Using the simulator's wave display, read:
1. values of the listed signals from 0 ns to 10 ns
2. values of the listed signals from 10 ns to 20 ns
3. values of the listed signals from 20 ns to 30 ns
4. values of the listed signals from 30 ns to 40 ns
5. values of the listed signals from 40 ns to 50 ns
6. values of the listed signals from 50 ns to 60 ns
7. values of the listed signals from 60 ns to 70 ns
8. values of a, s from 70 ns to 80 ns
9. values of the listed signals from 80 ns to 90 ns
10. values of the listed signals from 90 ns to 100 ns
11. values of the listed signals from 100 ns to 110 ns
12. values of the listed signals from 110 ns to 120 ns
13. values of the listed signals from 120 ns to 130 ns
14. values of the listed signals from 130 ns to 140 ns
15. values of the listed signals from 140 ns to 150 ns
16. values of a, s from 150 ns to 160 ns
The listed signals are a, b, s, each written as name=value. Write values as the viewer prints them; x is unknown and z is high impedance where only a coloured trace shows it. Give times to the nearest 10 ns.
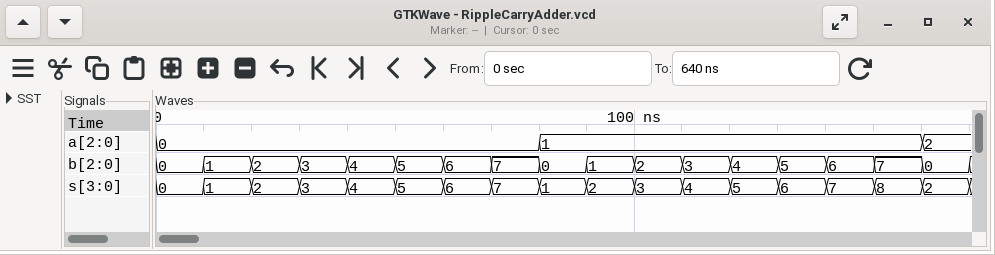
a=0, b=0, s=0
a=0, b=1, s=1
a=0, b=2, s=2
a=0, b=3, s=3
a=0, b=4, s=4
a=0, b=5, s=5
a=0, b=6, s=6
a=0, s=7
a=1, b=0, s=1
a=1, b=1, s=2
a=1, b=2, s=3
a=1, b=3, s=4
a=1, b=4, s=5
a=1, b=5, s=6
a=1, b=6, s=7
a=1, s=8
